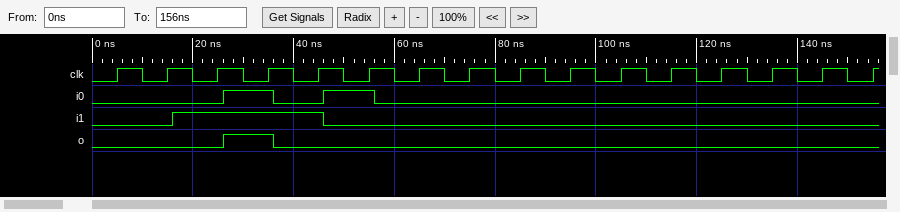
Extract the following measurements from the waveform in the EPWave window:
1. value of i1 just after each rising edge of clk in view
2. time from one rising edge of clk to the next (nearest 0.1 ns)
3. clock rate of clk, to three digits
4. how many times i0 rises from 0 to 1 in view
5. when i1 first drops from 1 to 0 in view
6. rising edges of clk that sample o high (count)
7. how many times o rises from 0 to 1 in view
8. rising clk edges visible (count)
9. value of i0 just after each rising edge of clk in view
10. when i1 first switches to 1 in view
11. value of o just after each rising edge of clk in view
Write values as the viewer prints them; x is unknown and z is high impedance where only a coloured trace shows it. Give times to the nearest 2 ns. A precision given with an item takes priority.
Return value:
0 0 1 1 1 0 0 0 0 0 0 0 0 0 0 0
10 ns
100 MHz
2
46 ns
1
1
16
0 0 0 1 0 1 0 0 0 0 0 0 0 0 0 0
16 ns
0 0 0 1 0 0 0 0 0 0 0 0 0 0 0 0
